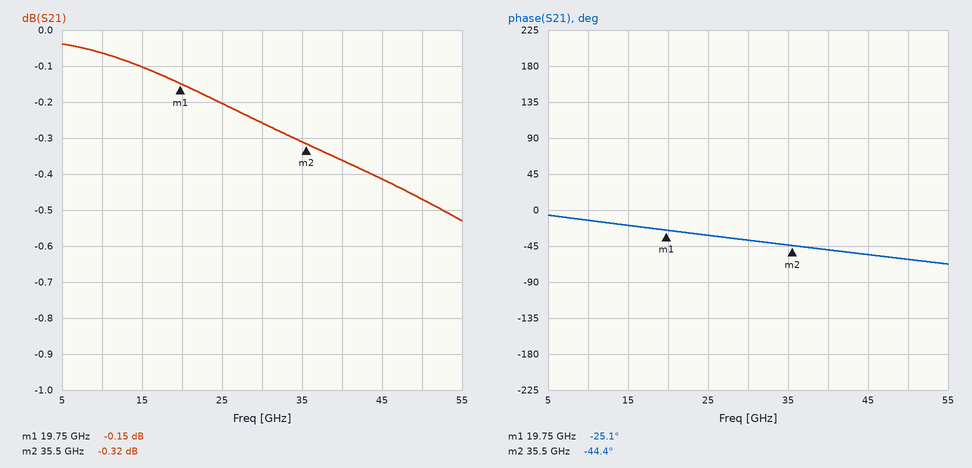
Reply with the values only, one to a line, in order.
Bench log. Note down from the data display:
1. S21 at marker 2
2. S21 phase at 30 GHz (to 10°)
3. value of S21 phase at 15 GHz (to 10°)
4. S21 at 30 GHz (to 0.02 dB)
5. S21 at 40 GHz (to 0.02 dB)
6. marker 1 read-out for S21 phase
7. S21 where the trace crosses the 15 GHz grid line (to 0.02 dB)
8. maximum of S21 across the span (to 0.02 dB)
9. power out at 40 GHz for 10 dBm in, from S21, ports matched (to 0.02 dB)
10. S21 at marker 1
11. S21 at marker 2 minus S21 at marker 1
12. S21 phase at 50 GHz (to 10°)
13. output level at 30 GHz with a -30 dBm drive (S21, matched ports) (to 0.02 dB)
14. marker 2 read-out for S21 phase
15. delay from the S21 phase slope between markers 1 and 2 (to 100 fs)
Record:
-0.32 dB
-40°
-20°
-0.26 dB
-0.36 dB
-25.1°
-0.10 dB
-0.04 dB
9.64 dBm
-0.15 dB
-0.17 dB
-60°
-30.26 dBm
-44.4°
3.4 ps
